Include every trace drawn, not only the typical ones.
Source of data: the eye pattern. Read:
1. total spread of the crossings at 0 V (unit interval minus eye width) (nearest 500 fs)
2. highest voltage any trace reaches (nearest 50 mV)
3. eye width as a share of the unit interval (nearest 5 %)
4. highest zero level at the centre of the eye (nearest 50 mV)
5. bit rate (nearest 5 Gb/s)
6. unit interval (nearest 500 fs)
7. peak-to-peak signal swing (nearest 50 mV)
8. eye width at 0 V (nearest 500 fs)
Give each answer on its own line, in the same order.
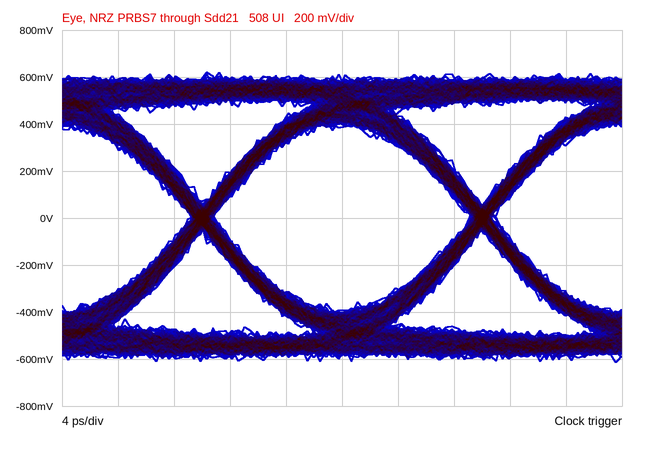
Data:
2.0 ps
600 mV
90 %
-400 mV
50 Gb/s
20.0 ps
1.25 V
18.0 ps
